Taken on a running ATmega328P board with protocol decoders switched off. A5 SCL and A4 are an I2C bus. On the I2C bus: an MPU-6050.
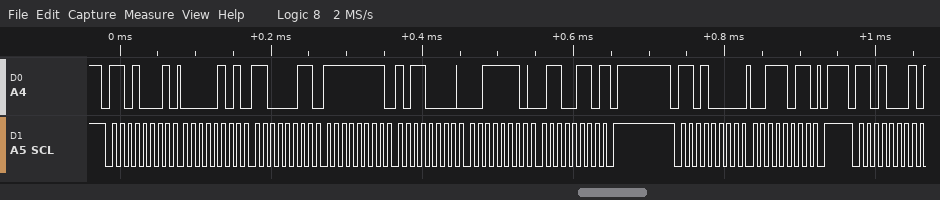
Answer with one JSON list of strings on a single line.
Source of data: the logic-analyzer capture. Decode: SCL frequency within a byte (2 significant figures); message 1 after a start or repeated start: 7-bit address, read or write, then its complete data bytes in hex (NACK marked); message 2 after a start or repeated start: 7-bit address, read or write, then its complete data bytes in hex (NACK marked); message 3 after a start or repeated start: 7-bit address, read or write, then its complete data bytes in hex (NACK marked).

["100 kHz", "0x68 read: 05 C3 FF B0 3E 66 NACK", "0x68 write: 3B", "0x68 read"]
